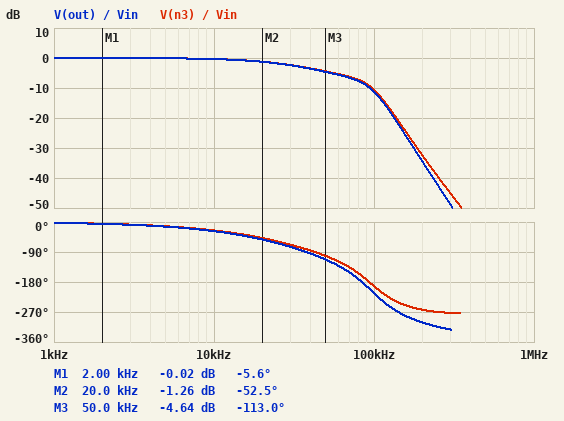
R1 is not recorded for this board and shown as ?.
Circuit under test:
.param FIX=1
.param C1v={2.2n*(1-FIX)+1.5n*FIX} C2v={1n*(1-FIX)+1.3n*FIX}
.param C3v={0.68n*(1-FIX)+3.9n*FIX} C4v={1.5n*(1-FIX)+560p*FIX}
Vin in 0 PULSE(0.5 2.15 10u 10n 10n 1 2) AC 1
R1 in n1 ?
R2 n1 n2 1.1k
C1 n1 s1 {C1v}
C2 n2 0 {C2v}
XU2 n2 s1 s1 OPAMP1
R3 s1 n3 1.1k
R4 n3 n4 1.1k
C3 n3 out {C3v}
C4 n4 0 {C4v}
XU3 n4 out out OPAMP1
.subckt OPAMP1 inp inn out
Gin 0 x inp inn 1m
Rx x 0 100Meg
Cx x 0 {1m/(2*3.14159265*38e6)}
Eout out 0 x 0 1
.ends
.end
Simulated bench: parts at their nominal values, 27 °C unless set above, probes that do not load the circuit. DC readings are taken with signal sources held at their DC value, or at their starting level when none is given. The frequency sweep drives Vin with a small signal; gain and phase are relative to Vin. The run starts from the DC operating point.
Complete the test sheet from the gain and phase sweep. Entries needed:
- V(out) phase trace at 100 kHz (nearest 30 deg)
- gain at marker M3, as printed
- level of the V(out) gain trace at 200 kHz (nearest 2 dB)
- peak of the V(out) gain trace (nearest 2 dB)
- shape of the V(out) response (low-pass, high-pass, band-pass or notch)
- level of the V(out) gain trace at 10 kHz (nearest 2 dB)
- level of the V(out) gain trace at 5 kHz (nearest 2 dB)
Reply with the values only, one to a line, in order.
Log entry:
-210 deg
-4.64 dB
-34 dB
0 dB
low-pass
0 dB
0 dB
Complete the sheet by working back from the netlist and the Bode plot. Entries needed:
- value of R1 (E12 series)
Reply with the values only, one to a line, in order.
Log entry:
3.9 kΩ
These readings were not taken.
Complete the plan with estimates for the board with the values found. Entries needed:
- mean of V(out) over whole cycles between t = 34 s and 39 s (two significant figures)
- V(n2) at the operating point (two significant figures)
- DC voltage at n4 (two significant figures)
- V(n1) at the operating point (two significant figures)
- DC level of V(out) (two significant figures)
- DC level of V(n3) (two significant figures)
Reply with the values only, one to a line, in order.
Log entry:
1.3 V
500 mV
500 mV
500 mV
500 mV
500 mV
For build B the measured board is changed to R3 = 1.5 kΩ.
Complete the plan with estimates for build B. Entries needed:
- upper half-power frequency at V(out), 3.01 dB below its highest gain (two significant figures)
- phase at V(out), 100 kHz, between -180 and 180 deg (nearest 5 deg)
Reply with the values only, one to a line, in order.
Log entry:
38 kHz
125 deg
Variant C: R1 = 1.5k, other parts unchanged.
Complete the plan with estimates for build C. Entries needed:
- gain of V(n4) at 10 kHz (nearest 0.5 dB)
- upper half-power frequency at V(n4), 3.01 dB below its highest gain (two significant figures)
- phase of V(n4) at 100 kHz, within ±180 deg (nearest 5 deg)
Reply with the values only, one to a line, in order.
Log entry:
0 dB
92 kHz
170 deg
